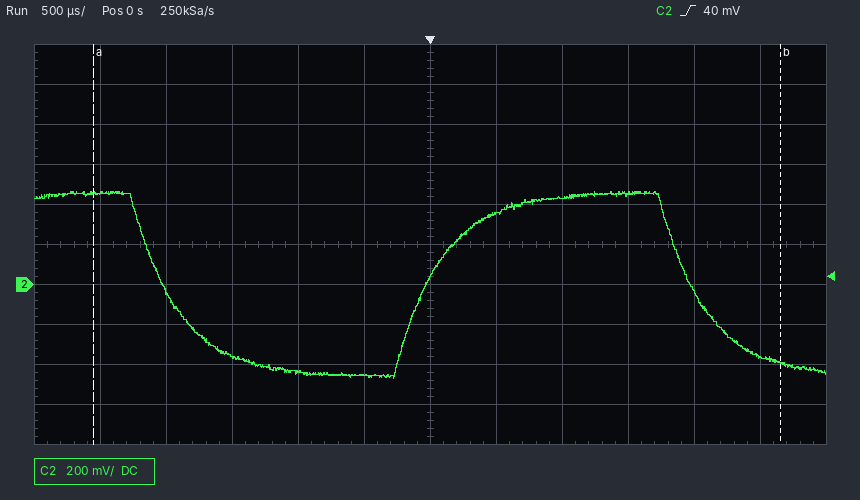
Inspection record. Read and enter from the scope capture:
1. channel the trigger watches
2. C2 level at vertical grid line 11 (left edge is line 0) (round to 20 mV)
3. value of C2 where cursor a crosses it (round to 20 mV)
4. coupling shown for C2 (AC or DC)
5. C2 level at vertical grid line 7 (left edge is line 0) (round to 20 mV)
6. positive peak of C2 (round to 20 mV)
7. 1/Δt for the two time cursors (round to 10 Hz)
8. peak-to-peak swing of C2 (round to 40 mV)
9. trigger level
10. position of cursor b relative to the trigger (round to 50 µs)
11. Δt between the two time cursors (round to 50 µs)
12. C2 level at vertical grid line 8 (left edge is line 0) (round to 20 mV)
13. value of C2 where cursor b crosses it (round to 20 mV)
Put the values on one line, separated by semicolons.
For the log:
C2; -360 mV; 460 mV; DC; 360 mV; 460 mV; 190 Hz; 920 mV; 40 mV; +2.65 ms; 5.20 ms; 440 mV; -400 mV
